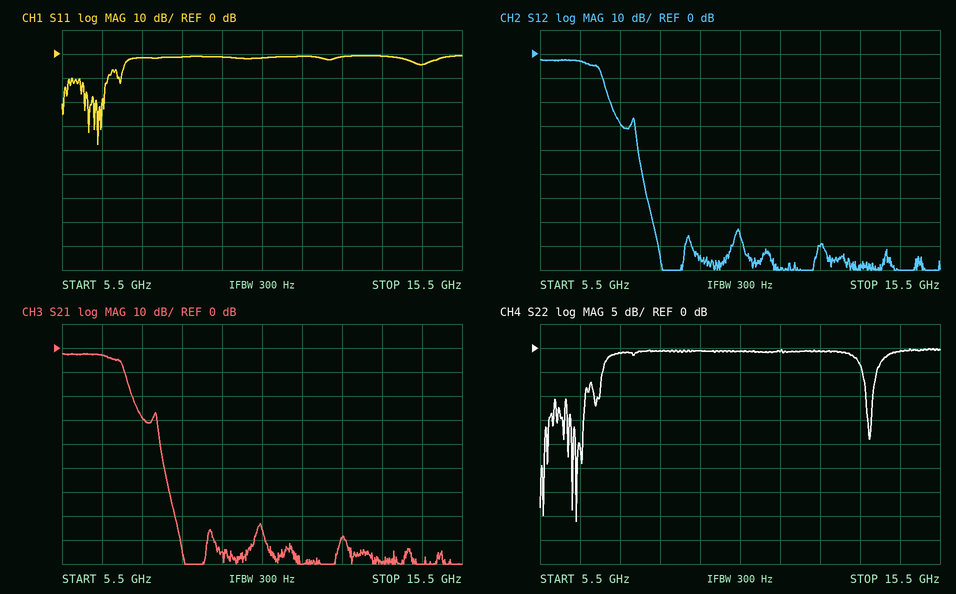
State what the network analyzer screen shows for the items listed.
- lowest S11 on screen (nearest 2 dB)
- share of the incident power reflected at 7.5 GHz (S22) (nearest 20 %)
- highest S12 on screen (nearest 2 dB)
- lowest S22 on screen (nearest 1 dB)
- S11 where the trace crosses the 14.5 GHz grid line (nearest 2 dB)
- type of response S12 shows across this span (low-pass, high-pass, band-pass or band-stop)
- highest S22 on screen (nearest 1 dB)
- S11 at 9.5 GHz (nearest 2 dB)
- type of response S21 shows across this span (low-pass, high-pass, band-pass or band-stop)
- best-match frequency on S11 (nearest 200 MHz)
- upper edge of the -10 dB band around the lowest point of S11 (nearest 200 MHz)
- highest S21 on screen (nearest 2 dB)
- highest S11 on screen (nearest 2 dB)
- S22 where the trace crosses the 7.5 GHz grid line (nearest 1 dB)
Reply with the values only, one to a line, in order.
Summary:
-38 dB
80 %
-2 dB
-36 dB
-4 dB
low-pass
0 dB
-2 dB
low-pass
6.4 GHz
6.6 GHz
-2 dB
0 dB
-1 dB
